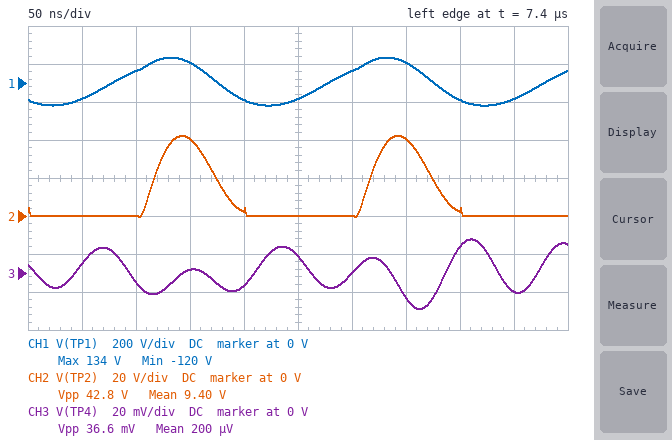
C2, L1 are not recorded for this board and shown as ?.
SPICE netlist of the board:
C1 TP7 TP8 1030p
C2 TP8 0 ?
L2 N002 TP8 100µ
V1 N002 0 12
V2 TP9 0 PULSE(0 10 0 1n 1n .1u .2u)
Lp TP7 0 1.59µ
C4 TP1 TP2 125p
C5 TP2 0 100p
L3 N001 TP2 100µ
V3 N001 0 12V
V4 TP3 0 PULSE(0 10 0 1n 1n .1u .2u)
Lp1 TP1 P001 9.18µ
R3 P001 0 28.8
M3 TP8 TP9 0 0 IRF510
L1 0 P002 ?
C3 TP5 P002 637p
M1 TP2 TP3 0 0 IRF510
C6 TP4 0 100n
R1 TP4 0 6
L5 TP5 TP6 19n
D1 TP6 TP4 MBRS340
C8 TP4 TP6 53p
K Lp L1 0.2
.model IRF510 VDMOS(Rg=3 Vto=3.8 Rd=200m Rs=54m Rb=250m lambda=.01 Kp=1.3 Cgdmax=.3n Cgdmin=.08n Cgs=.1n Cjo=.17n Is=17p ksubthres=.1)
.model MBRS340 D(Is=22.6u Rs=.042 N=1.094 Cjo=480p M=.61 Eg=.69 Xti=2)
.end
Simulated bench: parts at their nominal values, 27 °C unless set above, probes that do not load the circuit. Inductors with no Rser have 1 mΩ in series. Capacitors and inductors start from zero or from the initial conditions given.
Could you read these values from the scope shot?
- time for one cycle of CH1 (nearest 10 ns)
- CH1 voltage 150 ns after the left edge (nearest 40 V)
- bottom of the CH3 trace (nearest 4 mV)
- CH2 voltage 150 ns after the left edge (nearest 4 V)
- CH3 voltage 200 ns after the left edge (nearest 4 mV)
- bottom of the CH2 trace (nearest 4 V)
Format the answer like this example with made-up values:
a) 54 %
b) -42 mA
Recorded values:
a) 200 ns
b) 120 V
c) -20 mV
d) 40 V
e) -8 mV
f) 0 V
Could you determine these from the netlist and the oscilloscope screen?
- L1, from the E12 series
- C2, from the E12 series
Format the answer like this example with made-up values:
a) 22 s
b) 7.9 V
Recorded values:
a) 1.8 µH
b) 560 pF
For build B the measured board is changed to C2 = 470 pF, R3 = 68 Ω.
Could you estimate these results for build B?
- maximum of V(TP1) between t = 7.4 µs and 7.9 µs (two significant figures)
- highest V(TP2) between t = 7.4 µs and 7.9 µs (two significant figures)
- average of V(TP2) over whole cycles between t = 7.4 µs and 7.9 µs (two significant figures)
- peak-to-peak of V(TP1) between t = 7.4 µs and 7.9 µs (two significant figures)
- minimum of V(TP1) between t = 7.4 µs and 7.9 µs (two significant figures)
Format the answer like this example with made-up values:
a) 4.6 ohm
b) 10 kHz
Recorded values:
a) 72 V
b) 33 V
c) 12 V
d) 140 V
e) -72 V
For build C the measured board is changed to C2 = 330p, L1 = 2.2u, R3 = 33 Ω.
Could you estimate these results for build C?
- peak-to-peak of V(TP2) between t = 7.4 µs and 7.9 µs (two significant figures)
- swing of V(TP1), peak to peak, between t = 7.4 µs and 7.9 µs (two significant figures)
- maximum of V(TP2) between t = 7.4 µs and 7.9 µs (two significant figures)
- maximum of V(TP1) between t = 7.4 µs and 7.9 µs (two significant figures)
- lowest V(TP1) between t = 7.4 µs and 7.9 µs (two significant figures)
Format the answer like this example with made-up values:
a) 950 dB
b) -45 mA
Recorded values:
a) 41 V
b) 230 V
c) 40 V
d) 120 V
e) -110 V
